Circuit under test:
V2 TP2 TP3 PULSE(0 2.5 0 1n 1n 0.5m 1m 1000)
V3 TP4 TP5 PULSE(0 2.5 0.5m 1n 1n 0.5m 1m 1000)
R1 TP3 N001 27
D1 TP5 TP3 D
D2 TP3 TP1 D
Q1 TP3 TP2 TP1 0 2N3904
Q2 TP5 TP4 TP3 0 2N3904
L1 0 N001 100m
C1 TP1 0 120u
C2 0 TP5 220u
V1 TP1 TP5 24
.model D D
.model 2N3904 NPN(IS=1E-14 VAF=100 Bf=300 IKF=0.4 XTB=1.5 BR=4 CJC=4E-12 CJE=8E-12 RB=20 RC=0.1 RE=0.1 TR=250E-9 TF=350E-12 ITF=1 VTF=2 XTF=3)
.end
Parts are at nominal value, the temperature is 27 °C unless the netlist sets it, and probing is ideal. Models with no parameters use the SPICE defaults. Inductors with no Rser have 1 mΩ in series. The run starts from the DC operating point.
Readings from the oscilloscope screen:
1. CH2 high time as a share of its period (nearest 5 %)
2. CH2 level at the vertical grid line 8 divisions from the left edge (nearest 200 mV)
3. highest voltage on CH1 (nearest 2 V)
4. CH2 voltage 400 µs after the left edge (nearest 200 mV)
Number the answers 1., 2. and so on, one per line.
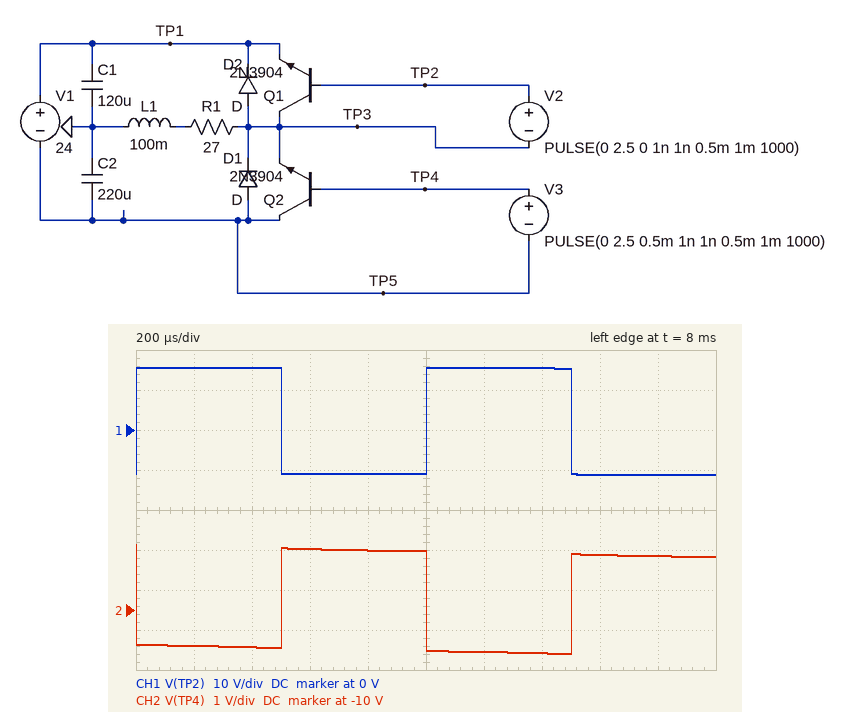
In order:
1. 50 %
2. -8.6 V
3. 16 V
4. -11.0 V
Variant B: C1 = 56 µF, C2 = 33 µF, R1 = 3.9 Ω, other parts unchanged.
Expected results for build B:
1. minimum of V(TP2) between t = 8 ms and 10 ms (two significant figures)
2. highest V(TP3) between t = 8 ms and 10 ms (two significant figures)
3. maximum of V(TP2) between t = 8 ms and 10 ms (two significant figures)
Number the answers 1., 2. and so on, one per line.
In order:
1. -14 V
2. 10 V
3. 13 V
